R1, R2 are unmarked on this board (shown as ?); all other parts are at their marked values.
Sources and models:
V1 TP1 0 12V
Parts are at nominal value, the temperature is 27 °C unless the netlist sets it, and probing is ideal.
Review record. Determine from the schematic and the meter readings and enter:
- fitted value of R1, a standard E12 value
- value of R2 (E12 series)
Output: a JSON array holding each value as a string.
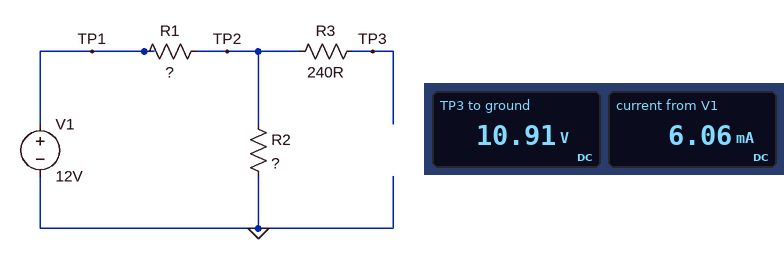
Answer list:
["180 Ω", "1.8 kΩ"]
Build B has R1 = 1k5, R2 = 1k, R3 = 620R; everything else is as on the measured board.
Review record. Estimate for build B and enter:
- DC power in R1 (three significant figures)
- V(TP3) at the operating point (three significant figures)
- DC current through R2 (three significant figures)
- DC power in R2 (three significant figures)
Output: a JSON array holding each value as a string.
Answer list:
["34.6 mW", "4.80 V", "4.80 mA", "23.0 mW"]
